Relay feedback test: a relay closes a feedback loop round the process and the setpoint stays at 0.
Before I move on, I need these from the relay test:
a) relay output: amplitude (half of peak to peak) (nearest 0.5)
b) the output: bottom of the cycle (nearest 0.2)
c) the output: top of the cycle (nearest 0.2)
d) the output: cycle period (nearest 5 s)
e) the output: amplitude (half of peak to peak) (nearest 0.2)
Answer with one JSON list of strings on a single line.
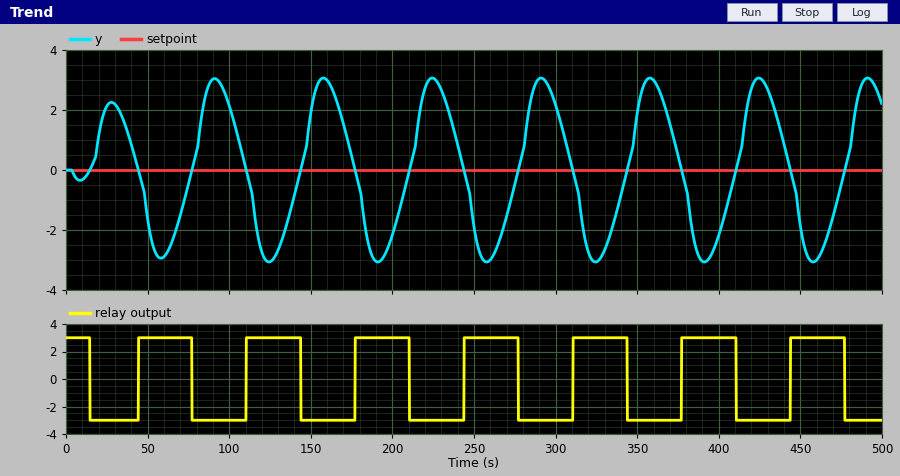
["3.0", "-3.0", "3.0", "65 s", "3.0"]
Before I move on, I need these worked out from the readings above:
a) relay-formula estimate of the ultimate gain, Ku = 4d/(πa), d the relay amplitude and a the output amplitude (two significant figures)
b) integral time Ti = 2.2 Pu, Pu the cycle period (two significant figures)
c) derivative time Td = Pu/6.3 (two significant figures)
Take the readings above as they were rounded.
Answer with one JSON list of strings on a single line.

["1.3", "140 s", "10 s"]
